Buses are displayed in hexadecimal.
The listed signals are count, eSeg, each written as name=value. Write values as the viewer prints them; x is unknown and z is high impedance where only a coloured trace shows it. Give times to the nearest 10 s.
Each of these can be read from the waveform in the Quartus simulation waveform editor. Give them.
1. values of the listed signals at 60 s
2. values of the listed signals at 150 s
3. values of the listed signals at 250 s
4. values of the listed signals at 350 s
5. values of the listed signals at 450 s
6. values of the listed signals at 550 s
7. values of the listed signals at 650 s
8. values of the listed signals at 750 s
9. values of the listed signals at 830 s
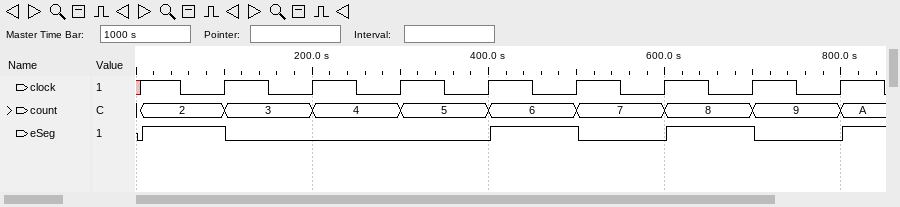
count=2, eSeg=1
count=3, eSeg=0
count=4, eSeg=0
count=5, eSeg=0
count=6, eSeg=1
count=7, eSeg=0
count=8, eSeg=1
count=9, eSeg=0
count=A, eSeg=1
